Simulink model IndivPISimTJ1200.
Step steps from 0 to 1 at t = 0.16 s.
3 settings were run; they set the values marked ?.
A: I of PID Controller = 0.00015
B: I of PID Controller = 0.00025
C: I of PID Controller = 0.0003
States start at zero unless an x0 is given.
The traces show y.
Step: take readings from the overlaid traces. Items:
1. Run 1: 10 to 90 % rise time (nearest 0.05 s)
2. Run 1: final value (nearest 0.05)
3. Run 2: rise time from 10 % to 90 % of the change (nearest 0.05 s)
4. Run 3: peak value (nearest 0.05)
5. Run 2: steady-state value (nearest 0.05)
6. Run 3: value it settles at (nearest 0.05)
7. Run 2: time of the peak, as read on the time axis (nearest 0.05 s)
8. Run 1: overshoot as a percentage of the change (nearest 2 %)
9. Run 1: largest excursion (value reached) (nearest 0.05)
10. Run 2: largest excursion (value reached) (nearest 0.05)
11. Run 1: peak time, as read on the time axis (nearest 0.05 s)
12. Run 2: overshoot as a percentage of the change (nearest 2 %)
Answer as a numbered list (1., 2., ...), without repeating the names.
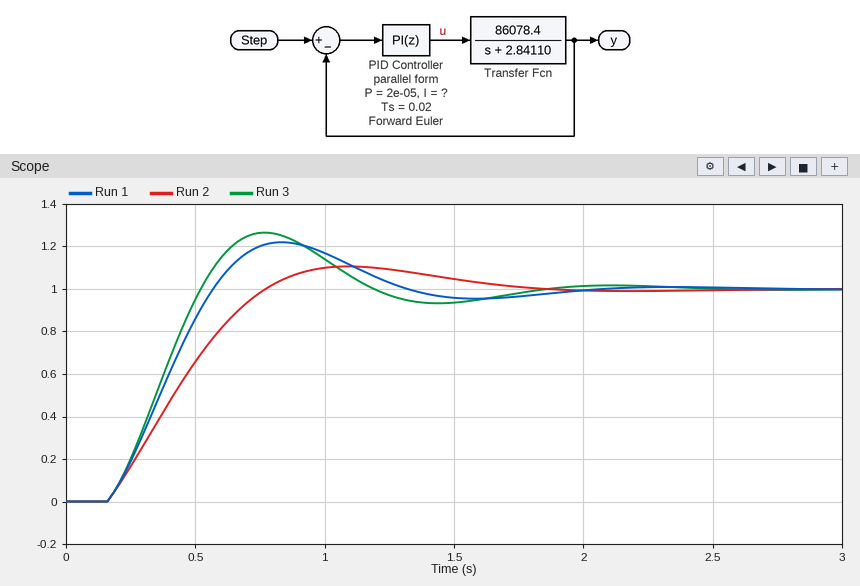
1. 0.30 s
2. 1.00
3. 0.45 s
4. 1.25
5. 1.00
6. 1.00
7. 1.10 s
8. 22 %
9. 1.20
10. 1.10
11. 0.85 s
12. 10 %
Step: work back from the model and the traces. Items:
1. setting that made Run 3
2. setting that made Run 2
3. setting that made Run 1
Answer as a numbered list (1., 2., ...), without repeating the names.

1. C
2. A
3. B
